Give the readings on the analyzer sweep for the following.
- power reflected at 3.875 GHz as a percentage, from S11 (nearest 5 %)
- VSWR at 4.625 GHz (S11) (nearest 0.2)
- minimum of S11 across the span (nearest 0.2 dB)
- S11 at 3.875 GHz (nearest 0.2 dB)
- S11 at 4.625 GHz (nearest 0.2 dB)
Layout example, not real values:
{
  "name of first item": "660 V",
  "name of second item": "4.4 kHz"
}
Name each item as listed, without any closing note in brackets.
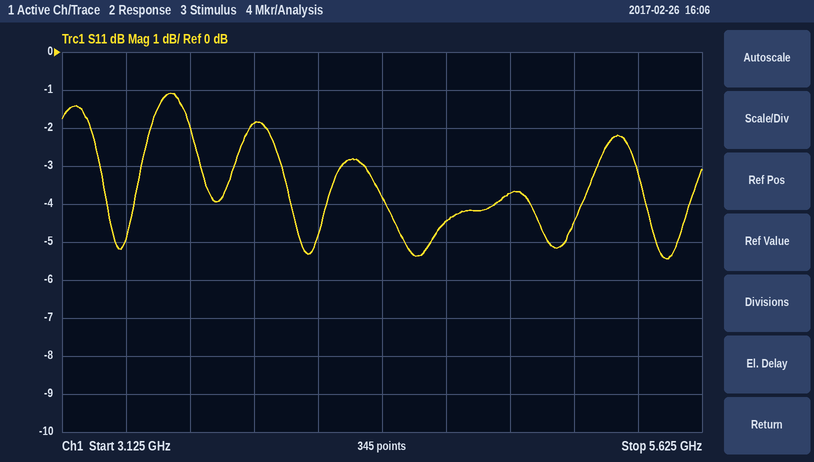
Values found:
{
  "power reflected at 3.875 GHz as a percentage, from S11": "65 %",
  "VSWR at 4.625 GHz (S11)": "4.0",
  "minimum of S11 across the span": "-5.4 dB",
  "S11 at 3.875 GHz": "-1.8 dB",
  "S11 at 4.625 GHz": "-4.4 dB"
}
